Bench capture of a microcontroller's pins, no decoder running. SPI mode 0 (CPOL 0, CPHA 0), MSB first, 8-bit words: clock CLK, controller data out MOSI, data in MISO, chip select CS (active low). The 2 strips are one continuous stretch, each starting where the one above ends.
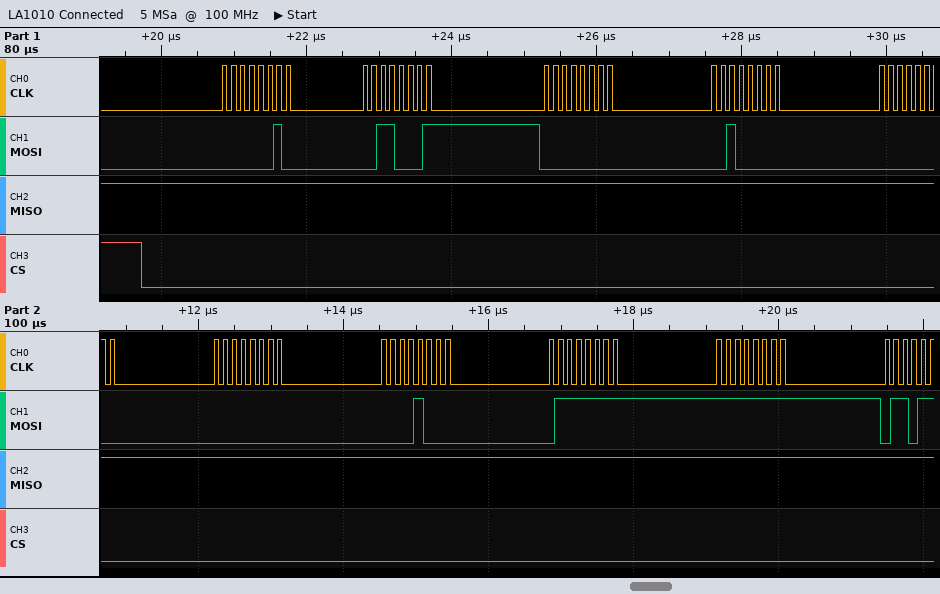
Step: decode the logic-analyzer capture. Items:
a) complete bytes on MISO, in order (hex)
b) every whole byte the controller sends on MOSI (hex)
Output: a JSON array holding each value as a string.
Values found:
["FF FF FF FF FF FF FF FF FF", "02 31 00 20 00 00 08 7F FF"]
